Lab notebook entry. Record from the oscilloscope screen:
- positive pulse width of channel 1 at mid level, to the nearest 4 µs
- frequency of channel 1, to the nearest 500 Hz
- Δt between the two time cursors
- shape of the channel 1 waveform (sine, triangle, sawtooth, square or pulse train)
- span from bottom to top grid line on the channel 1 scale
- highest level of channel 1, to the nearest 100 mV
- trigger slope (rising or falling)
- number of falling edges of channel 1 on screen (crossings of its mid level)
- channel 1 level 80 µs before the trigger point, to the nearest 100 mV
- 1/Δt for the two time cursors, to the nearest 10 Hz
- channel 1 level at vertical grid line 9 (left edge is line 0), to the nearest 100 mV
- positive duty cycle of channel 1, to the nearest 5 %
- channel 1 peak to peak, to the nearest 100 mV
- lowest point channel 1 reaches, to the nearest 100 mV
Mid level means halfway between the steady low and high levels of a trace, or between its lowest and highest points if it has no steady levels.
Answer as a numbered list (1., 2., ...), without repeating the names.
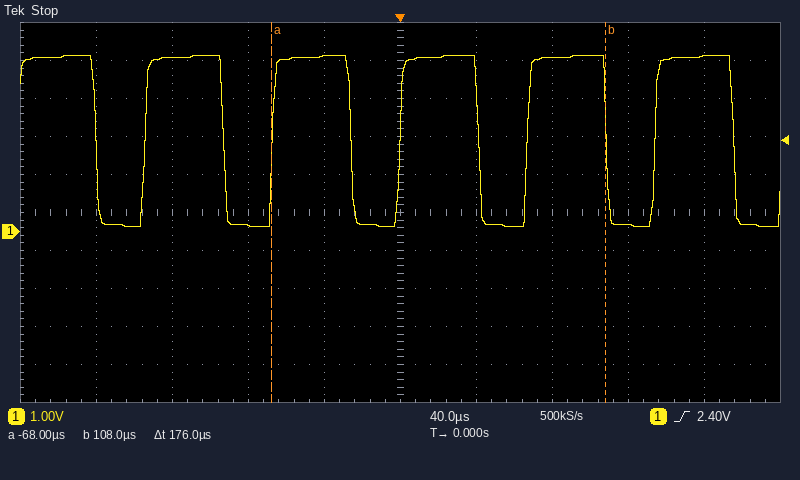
1. 40 µs
2. 15.0 kHz
3. 176 µs
4. pulse train
5. 10 V
6. 4.6 V
7. rising
8. 6
9. 200 mV
10. 5.68 kHz
11. 4.6 V
12. 60 %
13. 4.5 V
14. 100 mV
